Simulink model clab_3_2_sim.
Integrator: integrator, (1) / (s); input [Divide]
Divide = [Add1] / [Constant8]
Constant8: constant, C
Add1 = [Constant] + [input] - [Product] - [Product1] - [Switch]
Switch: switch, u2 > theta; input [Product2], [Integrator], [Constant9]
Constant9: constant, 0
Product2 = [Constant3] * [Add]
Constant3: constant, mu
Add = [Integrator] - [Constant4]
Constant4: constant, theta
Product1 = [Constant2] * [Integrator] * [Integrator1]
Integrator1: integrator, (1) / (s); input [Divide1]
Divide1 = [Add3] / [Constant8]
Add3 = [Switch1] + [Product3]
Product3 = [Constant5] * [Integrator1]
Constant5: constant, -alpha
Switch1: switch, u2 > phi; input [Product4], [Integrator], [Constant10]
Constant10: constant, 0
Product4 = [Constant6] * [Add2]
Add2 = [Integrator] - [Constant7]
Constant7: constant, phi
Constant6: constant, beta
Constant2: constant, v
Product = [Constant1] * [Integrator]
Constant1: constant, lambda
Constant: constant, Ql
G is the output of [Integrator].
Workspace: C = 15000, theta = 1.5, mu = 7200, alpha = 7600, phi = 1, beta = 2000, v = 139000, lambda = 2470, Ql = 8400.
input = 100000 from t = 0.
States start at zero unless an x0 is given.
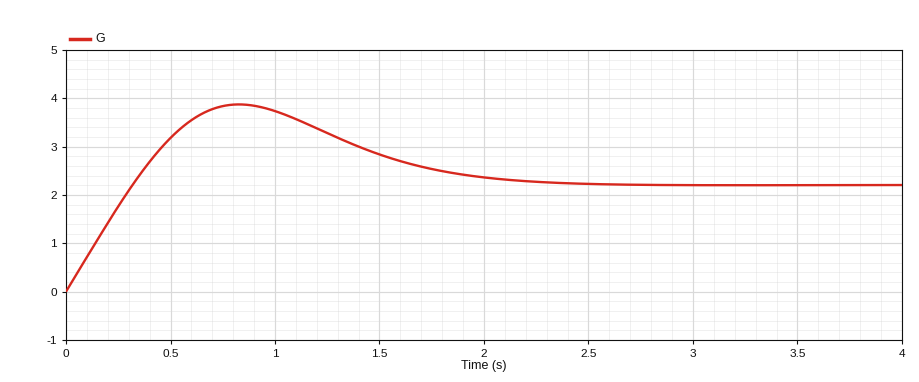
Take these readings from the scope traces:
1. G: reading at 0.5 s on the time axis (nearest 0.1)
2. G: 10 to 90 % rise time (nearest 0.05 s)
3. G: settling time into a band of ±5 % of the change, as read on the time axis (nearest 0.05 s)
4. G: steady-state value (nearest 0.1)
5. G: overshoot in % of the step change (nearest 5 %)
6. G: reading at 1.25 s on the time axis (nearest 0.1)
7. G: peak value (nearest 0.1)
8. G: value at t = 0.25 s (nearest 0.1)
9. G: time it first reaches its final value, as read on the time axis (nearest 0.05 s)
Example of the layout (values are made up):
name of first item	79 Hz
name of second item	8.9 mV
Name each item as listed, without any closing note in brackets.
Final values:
G: reading at 0.5 s on the time axis	3.2
G: 10 to 90 % rise time	0.25 s
G: settling time into a band of ±5 % of the change, as read on the time axis	2.10 s
G: steady-state value	2.2
G: overshoot in % of the step change	75 %
G: reading at 1.25 s on the time axis	3.3
G: peak value	3.9
G: value at t = 0.25 s	1.8
G: time it first reaches its final value, as read on the time axis	0.30 s
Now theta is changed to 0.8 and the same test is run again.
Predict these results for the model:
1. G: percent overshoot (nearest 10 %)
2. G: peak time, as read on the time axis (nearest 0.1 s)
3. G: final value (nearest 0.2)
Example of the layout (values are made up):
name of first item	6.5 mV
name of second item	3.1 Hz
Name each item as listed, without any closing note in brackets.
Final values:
G: percent overshoot	70 %
G: peak time, as read on the time axis	0.8 s
G: final value	2.2
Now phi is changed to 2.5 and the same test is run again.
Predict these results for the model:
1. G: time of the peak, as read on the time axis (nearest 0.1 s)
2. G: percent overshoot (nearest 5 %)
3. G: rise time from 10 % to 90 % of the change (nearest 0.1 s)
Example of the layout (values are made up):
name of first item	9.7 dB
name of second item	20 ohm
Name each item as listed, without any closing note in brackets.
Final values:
G: time of the peak, as read on the time axis	1.0 s
G: percent overshoot	45 %
G: rise time from 10 % to 90 % of the change	0.4 s
